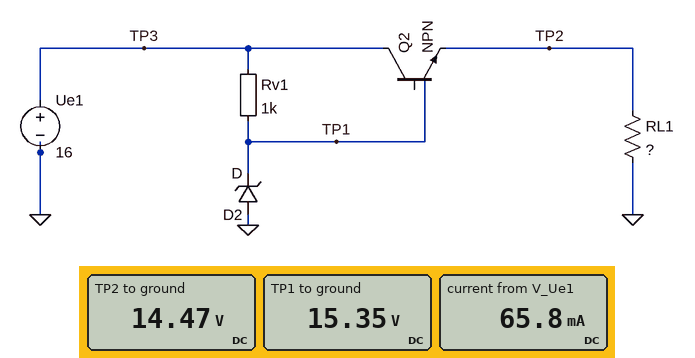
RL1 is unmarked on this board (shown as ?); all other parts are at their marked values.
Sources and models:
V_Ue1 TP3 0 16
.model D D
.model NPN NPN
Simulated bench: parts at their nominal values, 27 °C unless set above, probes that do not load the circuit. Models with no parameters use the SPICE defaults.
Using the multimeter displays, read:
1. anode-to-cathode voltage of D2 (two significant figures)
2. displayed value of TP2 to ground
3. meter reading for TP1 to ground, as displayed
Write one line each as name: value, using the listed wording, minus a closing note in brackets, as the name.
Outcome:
anode-to-cathode voltage of D2: -15 V
displayed value of TP2 to ground: 14.47 V
meter reading for TP1 to ground, as displayed: 15.35 V
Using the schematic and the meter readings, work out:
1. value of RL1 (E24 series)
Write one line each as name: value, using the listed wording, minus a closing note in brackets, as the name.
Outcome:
value of RL1: 220 Ω
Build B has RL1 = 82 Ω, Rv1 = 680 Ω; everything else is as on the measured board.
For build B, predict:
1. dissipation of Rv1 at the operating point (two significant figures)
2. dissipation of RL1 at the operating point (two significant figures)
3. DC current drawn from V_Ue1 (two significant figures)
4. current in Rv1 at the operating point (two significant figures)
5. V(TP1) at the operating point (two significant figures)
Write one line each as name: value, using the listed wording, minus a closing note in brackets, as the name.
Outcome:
dissipation of Rv1 at the operating point: 1.9 mW
dissipation of RL1 at the operating point: 2.4 W
DC current drawn from V_Ue1: 170 mA
current in Rv1 at the operating point: 1.7 mA
V(TP1) at the operating point: 15 V
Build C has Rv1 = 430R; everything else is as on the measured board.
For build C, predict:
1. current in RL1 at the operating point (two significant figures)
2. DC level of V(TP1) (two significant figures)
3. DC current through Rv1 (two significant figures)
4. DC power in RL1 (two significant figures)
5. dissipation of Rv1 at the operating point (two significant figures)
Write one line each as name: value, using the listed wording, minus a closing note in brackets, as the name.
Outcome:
current in RL1 at the operating point: 67 mA
DC level of V(TP1): 16 V
DC current through Rv1: 670 µA
DC power in RL1: 1.0 W
dissipation of Rv1 at the operating point: 190 µW
